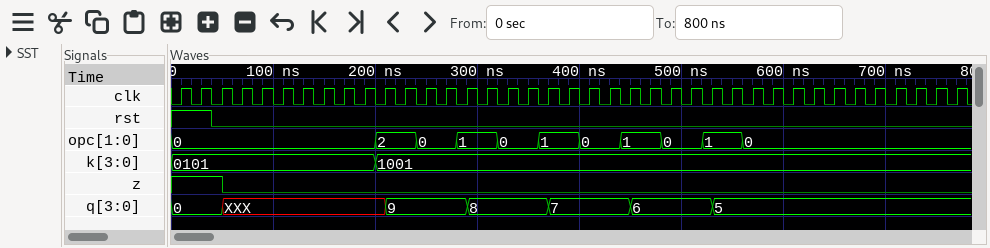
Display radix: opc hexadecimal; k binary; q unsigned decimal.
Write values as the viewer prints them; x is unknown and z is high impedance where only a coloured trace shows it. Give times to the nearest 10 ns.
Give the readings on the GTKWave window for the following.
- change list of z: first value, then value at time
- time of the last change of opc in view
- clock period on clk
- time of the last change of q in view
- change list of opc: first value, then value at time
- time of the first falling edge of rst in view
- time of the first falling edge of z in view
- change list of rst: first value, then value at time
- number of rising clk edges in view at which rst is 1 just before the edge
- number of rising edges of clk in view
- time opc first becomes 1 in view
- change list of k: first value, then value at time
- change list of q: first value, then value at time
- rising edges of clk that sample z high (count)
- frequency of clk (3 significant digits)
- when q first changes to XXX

1, 0 at 50 ns
560 ns
20 ns
530 ns
0, 2 at 200 ns, 0 at 240 ns, 1 at 280 ns, 0 at 320 ns, 1 at 360 ns, 0 at 400 ns, 1 at 440 ns, 0 at 480 ns, 1 at 520 ns, 0 at 560 ns
40 ns
50 ns
1, 0 at 40 ns
2
39
280 ns
0101, 1001 at 200 ns
0, XXX at 50 ns, 9 at 210 ns, 8 at 290 ns, 7 at 370 ns, 6 at 450 ns, 5 at 530 ns
3
50.0 MHz
50 ns
